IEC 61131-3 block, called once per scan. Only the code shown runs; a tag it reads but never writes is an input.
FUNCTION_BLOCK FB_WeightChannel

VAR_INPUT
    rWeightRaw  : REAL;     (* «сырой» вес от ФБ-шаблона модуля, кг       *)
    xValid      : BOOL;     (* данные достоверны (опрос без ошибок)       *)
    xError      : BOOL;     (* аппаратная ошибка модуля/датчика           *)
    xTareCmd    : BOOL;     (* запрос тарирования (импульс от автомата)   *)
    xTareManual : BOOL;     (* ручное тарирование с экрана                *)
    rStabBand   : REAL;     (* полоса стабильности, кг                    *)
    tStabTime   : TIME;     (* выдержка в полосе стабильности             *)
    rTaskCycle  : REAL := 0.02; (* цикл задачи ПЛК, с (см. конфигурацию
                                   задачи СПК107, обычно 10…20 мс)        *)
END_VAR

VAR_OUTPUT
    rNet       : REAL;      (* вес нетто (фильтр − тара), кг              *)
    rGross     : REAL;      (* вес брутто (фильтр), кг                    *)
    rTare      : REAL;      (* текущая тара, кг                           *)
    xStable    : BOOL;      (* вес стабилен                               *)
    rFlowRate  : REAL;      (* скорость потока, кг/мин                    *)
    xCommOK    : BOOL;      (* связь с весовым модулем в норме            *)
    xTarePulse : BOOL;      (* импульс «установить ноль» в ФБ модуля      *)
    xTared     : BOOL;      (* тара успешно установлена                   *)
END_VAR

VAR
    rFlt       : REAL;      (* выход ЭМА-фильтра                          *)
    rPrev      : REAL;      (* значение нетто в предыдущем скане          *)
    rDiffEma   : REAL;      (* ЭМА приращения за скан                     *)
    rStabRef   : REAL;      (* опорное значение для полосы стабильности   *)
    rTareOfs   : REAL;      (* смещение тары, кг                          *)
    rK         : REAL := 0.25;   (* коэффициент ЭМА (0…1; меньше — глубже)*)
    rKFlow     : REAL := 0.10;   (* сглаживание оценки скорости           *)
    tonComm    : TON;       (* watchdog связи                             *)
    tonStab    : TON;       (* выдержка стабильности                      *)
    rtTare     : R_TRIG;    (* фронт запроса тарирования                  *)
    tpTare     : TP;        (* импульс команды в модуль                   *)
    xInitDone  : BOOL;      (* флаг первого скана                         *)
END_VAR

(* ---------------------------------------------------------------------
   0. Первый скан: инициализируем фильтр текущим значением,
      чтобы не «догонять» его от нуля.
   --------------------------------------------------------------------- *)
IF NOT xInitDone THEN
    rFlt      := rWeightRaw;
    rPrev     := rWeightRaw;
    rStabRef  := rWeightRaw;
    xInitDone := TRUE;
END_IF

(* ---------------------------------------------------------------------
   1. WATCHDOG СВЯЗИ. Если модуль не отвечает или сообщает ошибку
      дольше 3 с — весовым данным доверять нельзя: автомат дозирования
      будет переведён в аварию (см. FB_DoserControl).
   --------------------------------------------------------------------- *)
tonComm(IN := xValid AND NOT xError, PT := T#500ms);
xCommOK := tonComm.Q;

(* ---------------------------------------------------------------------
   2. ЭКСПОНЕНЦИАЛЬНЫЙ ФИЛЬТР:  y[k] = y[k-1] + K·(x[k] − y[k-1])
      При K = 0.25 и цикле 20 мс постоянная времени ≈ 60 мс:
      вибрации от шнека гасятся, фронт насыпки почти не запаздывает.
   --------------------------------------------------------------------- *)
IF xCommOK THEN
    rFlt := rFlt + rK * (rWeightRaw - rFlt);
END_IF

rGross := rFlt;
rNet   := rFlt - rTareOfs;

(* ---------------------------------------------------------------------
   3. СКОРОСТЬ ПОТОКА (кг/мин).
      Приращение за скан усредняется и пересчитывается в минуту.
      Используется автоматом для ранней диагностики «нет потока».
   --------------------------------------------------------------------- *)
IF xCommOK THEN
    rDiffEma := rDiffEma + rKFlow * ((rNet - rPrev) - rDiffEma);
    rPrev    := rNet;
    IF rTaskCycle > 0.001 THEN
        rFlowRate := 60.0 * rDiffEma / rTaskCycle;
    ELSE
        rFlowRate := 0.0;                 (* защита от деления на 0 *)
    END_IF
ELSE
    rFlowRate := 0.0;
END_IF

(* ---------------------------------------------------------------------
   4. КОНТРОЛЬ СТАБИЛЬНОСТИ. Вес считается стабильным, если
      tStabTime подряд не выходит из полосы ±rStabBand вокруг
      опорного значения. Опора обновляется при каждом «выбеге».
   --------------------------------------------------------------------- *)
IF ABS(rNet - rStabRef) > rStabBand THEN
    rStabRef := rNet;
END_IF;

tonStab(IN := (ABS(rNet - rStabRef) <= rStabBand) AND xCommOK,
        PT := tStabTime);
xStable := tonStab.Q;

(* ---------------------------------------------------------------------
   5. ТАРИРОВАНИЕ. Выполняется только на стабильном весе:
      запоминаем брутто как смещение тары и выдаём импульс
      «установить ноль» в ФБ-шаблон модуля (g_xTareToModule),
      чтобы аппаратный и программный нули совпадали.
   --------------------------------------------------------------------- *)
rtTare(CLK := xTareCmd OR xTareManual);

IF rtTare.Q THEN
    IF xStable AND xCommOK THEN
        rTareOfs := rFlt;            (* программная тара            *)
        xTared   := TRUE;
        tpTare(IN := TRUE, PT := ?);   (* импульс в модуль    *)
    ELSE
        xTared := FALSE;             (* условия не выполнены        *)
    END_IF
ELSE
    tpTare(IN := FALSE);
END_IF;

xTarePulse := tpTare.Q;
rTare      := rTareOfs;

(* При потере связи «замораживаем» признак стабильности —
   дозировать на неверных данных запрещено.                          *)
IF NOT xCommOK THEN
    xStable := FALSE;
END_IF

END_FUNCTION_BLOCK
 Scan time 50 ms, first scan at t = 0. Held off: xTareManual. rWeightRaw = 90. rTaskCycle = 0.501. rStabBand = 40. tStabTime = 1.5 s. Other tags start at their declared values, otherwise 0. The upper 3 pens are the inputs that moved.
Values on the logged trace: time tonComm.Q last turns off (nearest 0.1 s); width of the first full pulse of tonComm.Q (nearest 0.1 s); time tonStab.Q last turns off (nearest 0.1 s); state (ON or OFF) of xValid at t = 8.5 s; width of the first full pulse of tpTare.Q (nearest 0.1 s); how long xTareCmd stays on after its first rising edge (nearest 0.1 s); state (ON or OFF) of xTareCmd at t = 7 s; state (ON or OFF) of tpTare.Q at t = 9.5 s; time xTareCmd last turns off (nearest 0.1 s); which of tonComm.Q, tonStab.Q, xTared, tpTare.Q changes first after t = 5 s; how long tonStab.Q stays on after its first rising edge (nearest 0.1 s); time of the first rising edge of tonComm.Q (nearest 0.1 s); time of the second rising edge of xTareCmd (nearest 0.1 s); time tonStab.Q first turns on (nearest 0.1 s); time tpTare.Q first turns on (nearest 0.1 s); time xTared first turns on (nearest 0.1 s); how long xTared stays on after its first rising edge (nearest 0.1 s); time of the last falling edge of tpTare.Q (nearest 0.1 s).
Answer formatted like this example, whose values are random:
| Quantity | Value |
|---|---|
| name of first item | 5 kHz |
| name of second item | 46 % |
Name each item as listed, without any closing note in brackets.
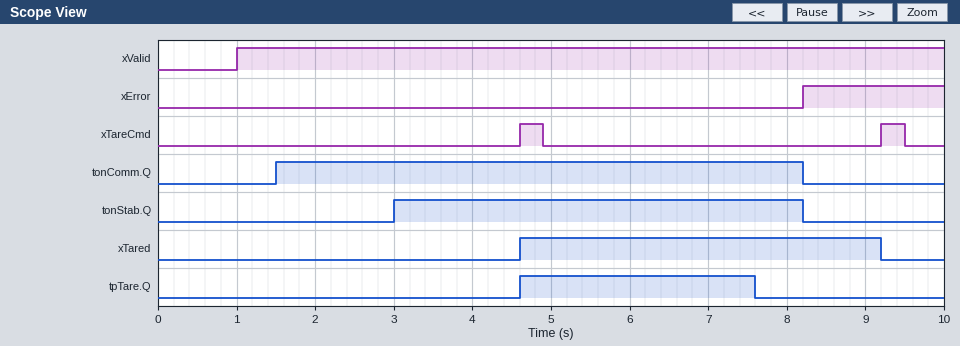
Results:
| Quantity | Value |
|---|---|
| time tonComm.Q last turns off | 8.2 s |
| width of the first full pulse of tonComm.Q | 6.7 s |
| time tonStab.Q last turns off | 8.2 s |
| state (ON or OFF) of xValid at t = 8.5 s | ON |
| width of the first full pulse of tpTare.Q | 3.0 s |
| how long xTareCmd stays on after its first rising edge | 0.3 s |
| state (ON or OFF) of xTareCmd at t = 7 s | OFF |
| state (ON or OFF) of tpTare.Q at t = 9.5 s | OFF |
| time xTareCmd last turns off | 9.5 s |
| which of tonComm.Q, tonStab.Q, xTared, tpTare.Q changes first after t = 5 s | tpTare.Q |
| how long tonStab.Q stays on after its first rising edge | 5.2 s |
| time of the first rising edge of tonComm.Q | 1.5 s |
| time of the second rising edge of xTareCmd | 9.2 s |
| time tonStab.Q first turns on | 3.0 s |
| time tpTare.Q first turns on | 4.6 s |
| time xTared first turns on | 4.6 s |
| how long xTared stays on after its first rising edge | 4.6 s |
| time of the last falling edge of tpTare.Q | 7.6 s |
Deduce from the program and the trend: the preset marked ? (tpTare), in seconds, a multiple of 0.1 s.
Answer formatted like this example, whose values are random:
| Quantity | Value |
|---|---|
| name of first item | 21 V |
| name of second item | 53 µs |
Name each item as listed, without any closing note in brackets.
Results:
| Quantity | Value |
|---|---|
| the preset marked ? (tpTare), in seconds, a multiple of 0.1 s | 3.0 s |
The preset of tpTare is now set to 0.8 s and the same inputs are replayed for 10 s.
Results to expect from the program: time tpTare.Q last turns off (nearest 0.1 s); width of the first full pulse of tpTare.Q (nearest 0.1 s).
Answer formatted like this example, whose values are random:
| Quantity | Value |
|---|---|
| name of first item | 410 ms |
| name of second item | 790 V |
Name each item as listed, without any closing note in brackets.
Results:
| Quantity | Value |
|---|---|
| time tpTare.Q last turns off | 5.4 s |
| width of the first full pulse of tpTare.Q | 0.8 s |
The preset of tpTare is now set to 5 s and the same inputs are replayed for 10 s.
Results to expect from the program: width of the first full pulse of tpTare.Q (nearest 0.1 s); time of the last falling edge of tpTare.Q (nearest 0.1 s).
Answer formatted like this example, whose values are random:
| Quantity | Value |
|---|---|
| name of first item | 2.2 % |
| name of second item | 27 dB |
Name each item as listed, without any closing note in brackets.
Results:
| Quantity | Value |
|---|---|
| width of the first full pulse of tpTare.Q | 5.0 s |
| time of the last falling edge of tpTare.Q | 9.6 s |
